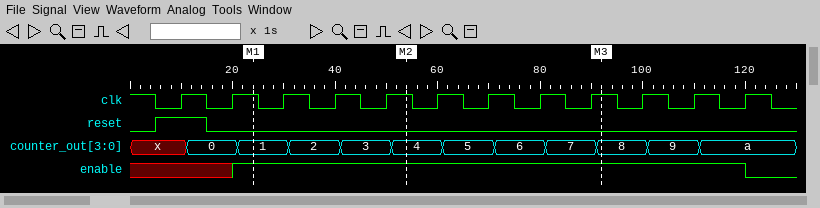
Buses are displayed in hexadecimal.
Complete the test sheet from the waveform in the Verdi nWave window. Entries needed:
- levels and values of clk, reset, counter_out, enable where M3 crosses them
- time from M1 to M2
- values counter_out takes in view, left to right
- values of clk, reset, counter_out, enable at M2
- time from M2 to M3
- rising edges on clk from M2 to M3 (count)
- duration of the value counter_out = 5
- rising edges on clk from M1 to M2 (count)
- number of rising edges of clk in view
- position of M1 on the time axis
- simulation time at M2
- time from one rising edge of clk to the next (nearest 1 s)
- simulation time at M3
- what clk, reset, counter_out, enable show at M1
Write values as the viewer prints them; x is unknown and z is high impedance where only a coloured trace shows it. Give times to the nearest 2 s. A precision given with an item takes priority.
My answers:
clk=1, reset=0, counter_out=8, enable=1
30 s
x, 0, 1, 2, 3, 4, 5, 6, 7, 8, 9, a
clk=1, reset=0, counter_out=4, enable=1
38 s
4
10 s
3
12
24 s
54 s
10 s
92 s
clk=1, reset=0, counter_out=1, enable=1
